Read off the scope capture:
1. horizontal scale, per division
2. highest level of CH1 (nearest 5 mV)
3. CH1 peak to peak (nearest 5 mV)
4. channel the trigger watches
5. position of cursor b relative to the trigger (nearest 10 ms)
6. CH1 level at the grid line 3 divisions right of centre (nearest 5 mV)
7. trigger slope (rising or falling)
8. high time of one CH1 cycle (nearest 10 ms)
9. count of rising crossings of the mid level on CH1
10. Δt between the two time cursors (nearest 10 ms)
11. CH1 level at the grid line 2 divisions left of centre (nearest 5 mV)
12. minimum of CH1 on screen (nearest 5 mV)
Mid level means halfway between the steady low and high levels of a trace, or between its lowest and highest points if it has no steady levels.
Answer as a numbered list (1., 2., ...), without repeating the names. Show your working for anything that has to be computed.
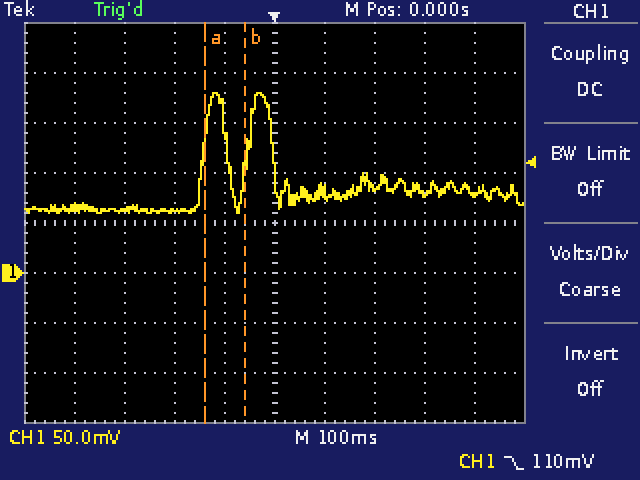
1. 100 ms
2. 180 mV
3. 180 mV − (60 mV) = 120 mV
4. CH1
5. -60 ms
6. 80 mV
7. falling
8. 50 ms
9. 2
10. 80 ms
11. 60 mV
12. 60 mV
